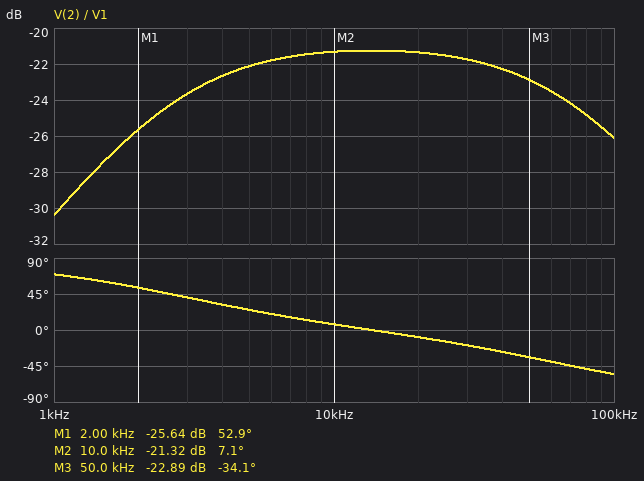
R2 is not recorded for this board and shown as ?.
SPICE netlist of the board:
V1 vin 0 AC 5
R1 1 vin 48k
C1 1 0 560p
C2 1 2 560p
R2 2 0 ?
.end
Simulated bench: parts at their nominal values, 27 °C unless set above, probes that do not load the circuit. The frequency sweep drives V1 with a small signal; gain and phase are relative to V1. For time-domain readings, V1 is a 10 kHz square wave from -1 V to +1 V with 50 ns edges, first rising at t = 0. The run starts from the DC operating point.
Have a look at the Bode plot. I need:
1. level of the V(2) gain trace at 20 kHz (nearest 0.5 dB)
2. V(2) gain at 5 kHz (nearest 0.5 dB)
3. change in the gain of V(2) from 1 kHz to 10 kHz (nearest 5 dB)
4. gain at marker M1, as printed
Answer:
-21.5 dB
-22.0 dB
10 dB
-25.64 dB
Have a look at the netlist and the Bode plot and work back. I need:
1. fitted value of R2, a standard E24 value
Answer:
9.1 kΩ
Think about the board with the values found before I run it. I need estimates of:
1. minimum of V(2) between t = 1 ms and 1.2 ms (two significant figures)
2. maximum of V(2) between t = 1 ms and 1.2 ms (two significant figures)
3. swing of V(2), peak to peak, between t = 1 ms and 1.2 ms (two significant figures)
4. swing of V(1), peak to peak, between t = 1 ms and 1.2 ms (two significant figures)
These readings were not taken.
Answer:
-110 mV
110 mV
220 mV
890 mV
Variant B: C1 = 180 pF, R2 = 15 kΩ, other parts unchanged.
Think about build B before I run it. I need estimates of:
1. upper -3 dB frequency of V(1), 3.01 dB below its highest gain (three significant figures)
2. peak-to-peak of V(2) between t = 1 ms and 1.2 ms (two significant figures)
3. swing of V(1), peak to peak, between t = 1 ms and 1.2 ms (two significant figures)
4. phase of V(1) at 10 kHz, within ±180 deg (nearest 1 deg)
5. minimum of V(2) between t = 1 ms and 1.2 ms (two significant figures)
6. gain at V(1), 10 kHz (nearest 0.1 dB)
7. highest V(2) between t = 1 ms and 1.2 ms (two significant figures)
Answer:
3.92 kHz
530 mV
1.2 V
-48 deg
-260 mV
-8.0 dB
260 mV
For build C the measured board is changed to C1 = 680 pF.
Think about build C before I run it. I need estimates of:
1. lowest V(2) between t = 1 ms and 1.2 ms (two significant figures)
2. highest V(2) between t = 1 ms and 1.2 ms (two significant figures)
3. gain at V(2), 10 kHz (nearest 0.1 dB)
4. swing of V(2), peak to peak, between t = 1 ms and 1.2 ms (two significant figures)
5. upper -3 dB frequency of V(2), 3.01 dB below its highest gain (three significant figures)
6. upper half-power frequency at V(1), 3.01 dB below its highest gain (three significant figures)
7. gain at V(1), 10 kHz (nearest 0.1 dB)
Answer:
-97 mV
97 mV
-22.1 dB
190 mV
64.2 kHz
2.58 kHz
-11.8 dB
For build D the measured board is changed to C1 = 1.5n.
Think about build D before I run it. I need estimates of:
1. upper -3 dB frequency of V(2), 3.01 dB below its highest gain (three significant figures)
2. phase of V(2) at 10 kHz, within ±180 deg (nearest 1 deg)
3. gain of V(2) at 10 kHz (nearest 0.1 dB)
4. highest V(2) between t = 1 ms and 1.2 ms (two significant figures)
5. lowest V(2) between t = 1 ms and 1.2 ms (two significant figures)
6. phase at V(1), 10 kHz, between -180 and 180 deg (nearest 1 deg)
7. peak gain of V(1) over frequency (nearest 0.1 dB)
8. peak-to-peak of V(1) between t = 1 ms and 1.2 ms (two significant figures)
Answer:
46.6 kHz
-4 deg
-26.2 dB
55 mV
-55 mV
-76 deg
0 dB
510 mV
